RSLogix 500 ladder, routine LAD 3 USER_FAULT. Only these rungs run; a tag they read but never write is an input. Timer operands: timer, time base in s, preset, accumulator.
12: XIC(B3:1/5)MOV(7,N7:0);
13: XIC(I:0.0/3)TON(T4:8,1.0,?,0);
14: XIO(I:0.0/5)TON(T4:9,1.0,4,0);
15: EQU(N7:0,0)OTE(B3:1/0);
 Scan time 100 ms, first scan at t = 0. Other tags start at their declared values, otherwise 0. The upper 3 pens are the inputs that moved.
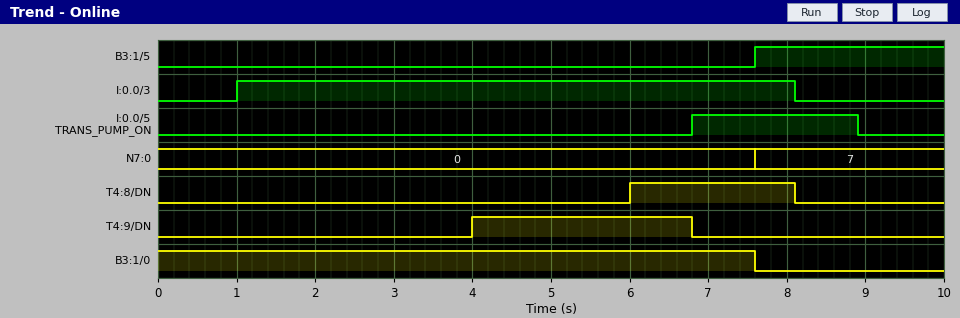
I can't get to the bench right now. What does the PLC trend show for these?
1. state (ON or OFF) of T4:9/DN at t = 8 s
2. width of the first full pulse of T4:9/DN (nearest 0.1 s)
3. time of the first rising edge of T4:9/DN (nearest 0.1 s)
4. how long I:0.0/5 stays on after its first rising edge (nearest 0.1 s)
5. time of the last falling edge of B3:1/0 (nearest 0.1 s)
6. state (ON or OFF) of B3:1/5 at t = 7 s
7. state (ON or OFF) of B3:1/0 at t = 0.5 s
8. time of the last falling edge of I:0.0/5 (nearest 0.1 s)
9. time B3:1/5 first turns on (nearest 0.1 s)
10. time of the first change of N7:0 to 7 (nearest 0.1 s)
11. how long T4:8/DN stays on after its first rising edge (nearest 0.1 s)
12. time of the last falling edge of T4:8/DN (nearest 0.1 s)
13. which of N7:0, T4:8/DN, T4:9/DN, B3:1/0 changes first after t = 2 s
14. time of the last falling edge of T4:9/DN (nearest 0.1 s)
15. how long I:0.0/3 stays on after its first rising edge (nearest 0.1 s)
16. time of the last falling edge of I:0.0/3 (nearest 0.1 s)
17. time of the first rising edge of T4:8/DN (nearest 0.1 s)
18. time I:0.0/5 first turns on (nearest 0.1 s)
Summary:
OFF
2.8 s
4.0 s
2.1 s
7.6 s
OFF
ON
8.9 s
7.6 s
7.6 s
2.1 s
8.1 s
T4:9/DN
6.8 s
7.1 s
8.1 s
6.0 s
6.8 s
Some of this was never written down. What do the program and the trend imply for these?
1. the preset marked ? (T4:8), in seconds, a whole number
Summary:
5 s
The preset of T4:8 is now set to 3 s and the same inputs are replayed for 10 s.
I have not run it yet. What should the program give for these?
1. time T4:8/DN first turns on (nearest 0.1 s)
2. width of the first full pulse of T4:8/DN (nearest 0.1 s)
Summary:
4.0 s
4.1 s
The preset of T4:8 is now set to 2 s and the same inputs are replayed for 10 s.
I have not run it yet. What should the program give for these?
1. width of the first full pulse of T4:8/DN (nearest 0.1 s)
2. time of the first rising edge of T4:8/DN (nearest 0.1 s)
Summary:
5.1 s
3.0 s
